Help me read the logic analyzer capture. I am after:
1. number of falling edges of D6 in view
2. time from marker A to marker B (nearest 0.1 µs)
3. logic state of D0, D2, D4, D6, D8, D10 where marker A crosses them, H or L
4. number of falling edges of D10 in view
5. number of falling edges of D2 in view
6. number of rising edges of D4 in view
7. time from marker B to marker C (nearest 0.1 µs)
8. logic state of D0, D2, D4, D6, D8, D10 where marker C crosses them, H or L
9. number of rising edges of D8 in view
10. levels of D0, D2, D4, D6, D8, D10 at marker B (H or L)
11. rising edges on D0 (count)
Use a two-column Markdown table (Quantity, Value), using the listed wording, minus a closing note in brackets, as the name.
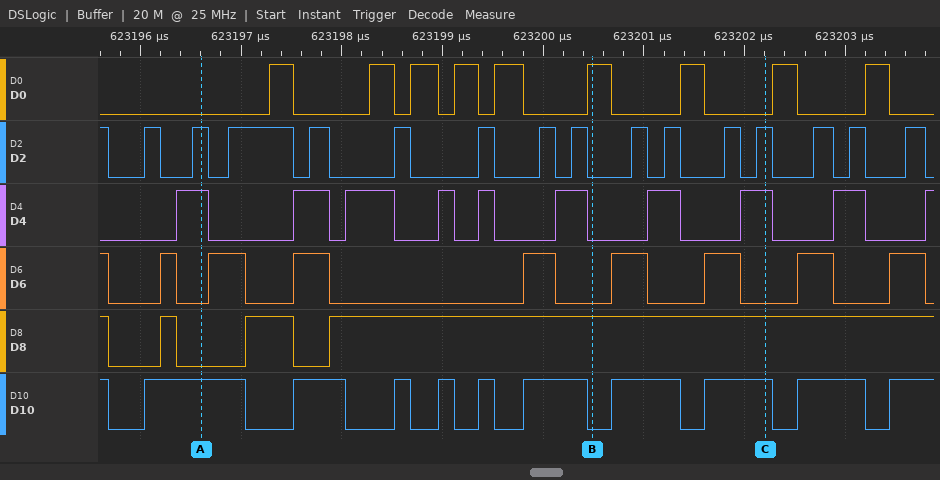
| Quantity | Value |
|---|---|
| number of falling edges of D6 in view | 9 |
| time from marker A to marker B | 3.9 µs |
| logic state of D0, D2, D4, D6, D8, D10 where marker A crosses them, H or L | D0=L, D2=H, D4=H, D6=L, D8=L, D10=H |
| number of falling edges of D10 in view | 10 |
| number of falling edges of D2 in view | 16 |
| number of rising edges of D4 in view | 10 |
| time from marker B to marker C | 1.7 µs |
| logic state of D0, D2, D4, D6, D8, D10 where marker C crosses them, H or L | D0=L, D2=H, D4=H, D6=L, D8=H, D10=H |
| number of rising edges of D8 in view | 3 |
| levels of D0, D2, D4, D6, D8, D10 at marker B | D0=H, D2=L, D4=L, D6=L, D8=H, D10=L |
| rising edges on D0 | 9 |
